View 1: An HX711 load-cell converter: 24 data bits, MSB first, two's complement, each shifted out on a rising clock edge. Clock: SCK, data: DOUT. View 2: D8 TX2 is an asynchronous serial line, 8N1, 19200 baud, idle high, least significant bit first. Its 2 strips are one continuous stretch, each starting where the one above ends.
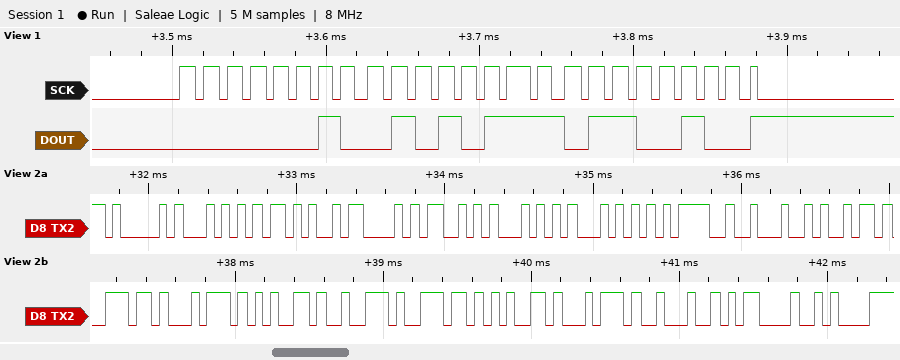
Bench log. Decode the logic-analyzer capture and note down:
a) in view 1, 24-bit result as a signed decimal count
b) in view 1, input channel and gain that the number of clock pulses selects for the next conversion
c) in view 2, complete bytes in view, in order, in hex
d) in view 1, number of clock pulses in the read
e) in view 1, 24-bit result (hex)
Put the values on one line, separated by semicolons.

153444; channel A, gain 128; 41 54 2B 43 53 54 54 3D 22 69 6E 74 65 72 6E 65 74 22 0D 0A; 25; 0x025764
